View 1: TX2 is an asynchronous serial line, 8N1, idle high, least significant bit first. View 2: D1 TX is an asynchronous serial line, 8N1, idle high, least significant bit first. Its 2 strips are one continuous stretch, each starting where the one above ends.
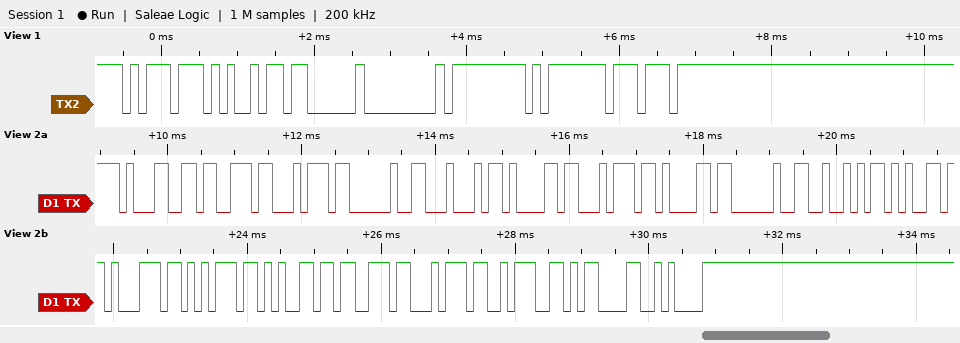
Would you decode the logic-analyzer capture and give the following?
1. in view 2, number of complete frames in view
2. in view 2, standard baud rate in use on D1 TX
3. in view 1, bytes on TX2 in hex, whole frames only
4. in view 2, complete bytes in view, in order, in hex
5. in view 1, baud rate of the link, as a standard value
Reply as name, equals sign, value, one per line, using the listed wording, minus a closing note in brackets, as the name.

in view 2, number of complete frames in view = 19
in view 2, standard baud rate in use on D1 TX = 9600 baud
in view 1, bytes on TX2 in hex, whole frames only = DD A5 03 00 FF FD 77
in view 2, complete bytes in view, in order, in hex = 0x31 0x73 0x74 0x20 0x44 0x61 0x74 0x61 0x20 0x52 0x65 0x71 0x75 0x65 0x73 0x74 0x3A 0x0D 0x0A
in view 1, baud rate of the link, as a standard value = 9600 baud
